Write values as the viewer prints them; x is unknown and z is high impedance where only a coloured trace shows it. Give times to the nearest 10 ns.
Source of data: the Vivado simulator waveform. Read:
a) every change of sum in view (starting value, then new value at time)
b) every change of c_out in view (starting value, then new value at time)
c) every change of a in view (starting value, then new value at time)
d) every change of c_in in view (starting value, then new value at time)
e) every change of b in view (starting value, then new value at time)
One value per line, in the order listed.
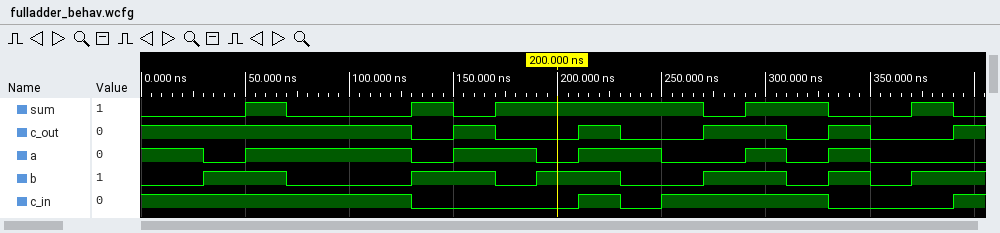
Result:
0, 1 at 50 ns, 0 at 70 ns, 1 at 130 ns, 0 at 150 ns, 1 at 170 ns, 0 at 270 ns, 1 at 290 ns, 0 at 330 ns, 1 at 370 ns, 0 at 390 ns
1, 0 at 130 ns, 1 at 150 ns, 0 at 170 ns, 1 at 210 ns, 0 at 230 ns, 1 at 270 ns, 0 at 310 ns, 1 at 330 ns, 0 at 350 ns, 1 at 390 ns
1, 0 at 30 ns, 1 at 50 ns, 0 at 130 ns, 1 at 150 ns, 0 at 190 ns, 1 at 210 ns, 0 at 250 ns, 1 at 290 ns, 0 at 310 ns, 1 at 330 ns, 0 at 350 ns
1, 0 at 130 ns, 1 at 210 ns, 0 at 230 ns, 1 at 250 ns, 0 at 330 ns, 1 at 390 ns
0, 1 at 30 ns, 0 at 70 ns, 1 at 130 ns, 0 at 170 ns, 1 at 190 ns, 0 at 230 ns, 1 at 270 ns, 0 at 310 ns, 1 at 330 ns, 0 at 350 ns, 1 at 370 ns
